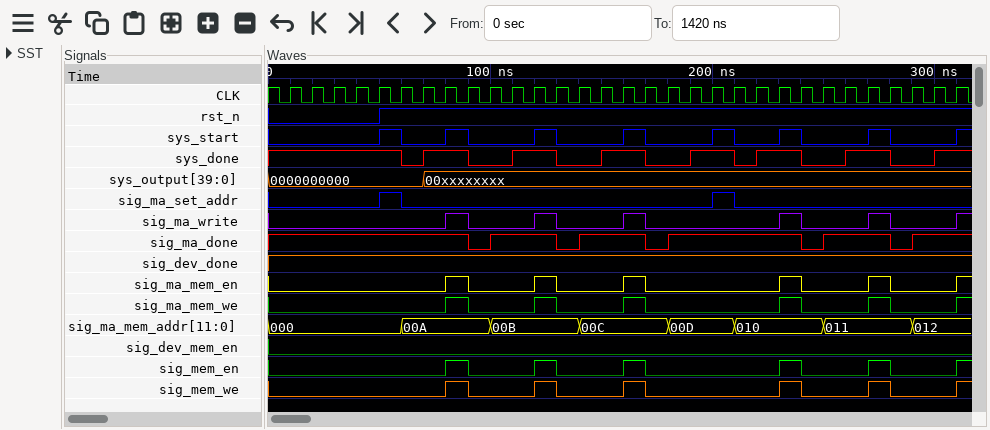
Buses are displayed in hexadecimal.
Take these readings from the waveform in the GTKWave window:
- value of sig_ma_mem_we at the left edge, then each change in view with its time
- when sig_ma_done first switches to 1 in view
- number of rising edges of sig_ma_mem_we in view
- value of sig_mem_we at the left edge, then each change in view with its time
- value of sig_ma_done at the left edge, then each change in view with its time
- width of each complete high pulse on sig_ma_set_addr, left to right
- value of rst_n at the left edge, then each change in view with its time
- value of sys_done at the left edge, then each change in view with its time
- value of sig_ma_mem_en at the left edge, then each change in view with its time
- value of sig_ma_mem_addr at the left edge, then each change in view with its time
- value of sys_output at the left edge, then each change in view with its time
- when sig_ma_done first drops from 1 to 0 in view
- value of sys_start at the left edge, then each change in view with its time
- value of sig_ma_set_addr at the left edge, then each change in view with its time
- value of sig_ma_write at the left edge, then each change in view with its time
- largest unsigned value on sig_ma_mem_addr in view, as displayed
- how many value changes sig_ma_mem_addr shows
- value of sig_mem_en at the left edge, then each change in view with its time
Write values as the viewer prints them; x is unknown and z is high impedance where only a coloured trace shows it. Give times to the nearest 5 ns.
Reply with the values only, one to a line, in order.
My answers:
0, 1 at 80 ns, 0 at 90 ns, 1 at 120 ns, 0 at 130 ns, 1 at 160 ns, 0 at 170 ns, 1 at 230 ns, 0 at 240 ns, 1 at 270 ns, 0 at 280 ns, 1 at 310 ns
100 ns
6
0, 1 at 80 ns, 0 at 90 ns, 1 at 120 ns, 0 at 130 ns, 1 at 160 ns, 0 at 170 ns, 1 at 230 ns, 0 at 240 ns, 1 at 270 ns, 0 at 280 ns, 1 at 310 ns
1, 0 at 90 ns, 1 at 100 ns, 0 at 130 ns, 1 at 140 ns, 0 at 170 ns, 1 at 180 ns, 0 at 240 ns, 1 at 250 ns, 0 at 280 ns, 1 at 290 ns
10 ns, 10 ns
0, 1 at 50 ns
1, 0 at 60 ns, 1 at 70 ns, 0 at 90 ns, 1 at 110 ns, 0 at 130 ns, 1 at 150 ns, 0 at 170 ns, 1 at 190 ns, 0 at 210 ns, 1 at 220 ns, 0 at 240 ns, 1 at 260 ns, 0 at 280 ns, 1 at 300 ns
0, 1 at 80 ns, 0 at 90 ns, 1 at 120 ns, 0 at 130 ns, 1 at 160 ns, 0 at 170 ns, 1 at 230 ns, 0 at 240 ns, 1 at 270 ns, 0 at 280 ns, 1 at 310 ns
000, 00A at 60 ns, 00B at 100 ns, 00C at 140 ns, 00D at 180 ns, 010 at 210 ns, 011 at 250 ns, 012 at 290 ns
0000000000, 00xxxxxxxx at 70 ns
90 ns
0, 1 at 50 ns, 0 at 60 ns, 1 at 80 ns, 0 at 90 ns, 1 at 120 ns, 0 at 130 ns, 1 at 160 ns, 0 at 170 ns, 1 at 200 ns, 0 at 210 ns, 1 at 230 ns, 0 at 240 ns, 1 at 270 ns, 0 at 280 ns, 1 at 310 ns
0, 1 at 50 ns, 0 at 60 ns, 1 at 200 ns, 0 at 210 ns
0, 1 at 80 ns, 0 at 90 ns, 1 at 120 ns, 0 at 130 ns, 1 at 160 ns, 0 at 170 ns, 1 at 230 ns, 0 at 240 ns, 1 at 270 ns, 0 at 280 ns, 1 at 310 ns
012
7
0, 1 at 80 ns, 0 at 90 ns, 1 at 120 ns, 0 at 130 ns, 1 at 160 ns, 0 at 170 ns, 1 at 230 ns, 0 at 240 ns, 1 at 270 ns, 0 at 280 ns, 1 at 310 ns
